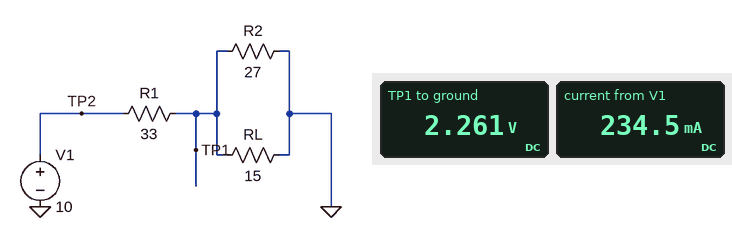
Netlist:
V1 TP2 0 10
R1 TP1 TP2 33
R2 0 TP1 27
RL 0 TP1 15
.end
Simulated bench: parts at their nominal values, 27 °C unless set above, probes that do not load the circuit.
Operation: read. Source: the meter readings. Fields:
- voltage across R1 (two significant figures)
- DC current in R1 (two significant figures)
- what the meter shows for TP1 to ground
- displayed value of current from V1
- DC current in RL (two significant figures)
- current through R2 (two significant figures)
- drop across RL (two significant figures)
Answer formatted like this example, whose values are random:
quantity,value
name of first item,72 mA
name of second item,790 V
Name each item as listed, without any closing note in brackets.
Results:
quantity,value
voltage across R1,7.7 V
DC current in R1,230 mA
what the meter shows for TP1 to ground,2.261 V
displayed value of current from V1,234.5 mA
DC current in RL,150 mA
current through R2,84 mA
drop across RL,2.3 V
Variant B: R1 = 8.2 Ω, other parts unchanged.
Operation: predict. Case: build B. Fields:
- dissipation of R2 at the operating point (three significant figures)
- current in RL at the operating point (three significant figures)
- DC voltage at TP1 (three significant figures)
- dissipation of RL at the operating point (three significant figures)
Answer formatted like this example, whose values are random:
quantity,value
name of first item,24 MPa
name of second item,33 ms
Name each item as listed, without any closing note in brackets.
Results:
quantity,value
dissipation of R2 at the operating point,1.08 W
current in RL at the operating point,360 mA
DC voltage at TP1,5.40 V
dissipation of RL at the operating point,1.95 W
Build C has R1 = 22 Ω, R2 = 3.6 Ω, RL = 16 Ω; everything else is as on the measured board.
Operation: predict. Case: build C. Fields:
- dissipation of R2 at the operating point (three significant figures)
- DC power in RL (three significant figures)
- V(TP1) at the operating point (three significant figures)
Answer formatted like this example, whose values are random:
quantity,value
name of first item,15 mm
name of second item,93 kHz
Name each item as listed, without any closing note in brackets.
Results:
quantity,value
dissipation of R2 at the operating point,386 mW
DC power in RL,86.8 mW
V(TP1) at the operating point,1.18 V
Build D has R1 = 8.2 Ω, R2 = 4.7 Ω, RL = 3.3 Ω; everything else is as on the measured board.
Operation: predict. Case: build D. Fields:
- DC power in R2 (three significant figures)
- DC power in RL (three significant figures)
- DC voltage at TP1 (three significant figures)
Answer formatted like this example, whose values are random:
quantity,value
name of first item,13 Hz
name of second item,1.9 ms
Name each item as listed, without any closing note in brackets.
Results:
quantity,value
DC power in R2,778 mW
DC power in RL,1.11 W
DC voltage at TP1,1.91 V
